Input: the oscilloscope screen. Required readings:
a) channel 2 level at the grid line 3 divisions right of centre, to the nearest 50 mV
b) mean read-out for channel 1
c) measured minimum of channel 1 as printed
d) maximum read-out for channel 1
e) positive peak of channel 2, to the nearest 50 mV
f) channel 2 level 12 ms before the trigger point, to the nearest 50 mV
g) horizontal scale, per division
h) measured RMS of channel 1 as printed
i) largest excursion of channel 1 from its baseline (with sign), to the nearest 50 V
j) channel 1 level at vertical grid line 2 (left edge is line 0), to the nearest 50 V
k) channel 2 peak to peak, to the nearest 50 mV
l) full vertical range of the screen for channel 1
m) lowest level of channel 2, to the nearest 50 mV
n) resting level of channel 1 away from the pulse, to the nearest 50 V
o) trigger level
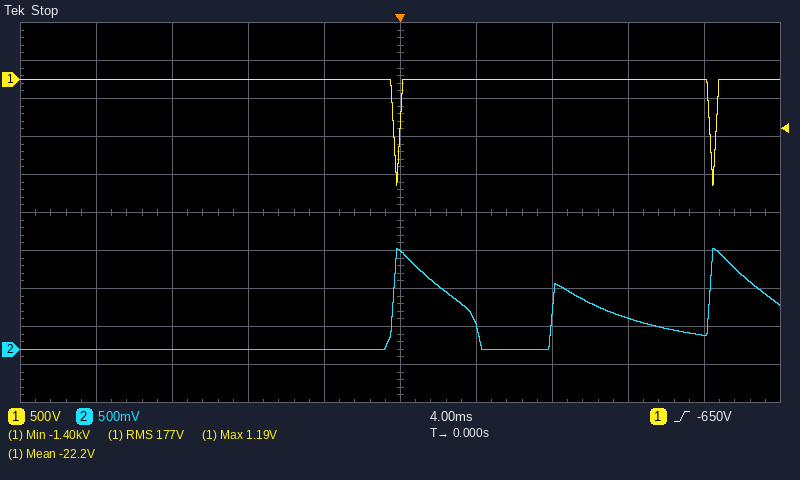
400 mV
-22.2 V
-1.40 kV
1.19 V
1.35 V
0 mV
4 ms
177 V
-1.40 kV
0 V
1.35 V
5 kV
0 mV
0 V
-650 V
